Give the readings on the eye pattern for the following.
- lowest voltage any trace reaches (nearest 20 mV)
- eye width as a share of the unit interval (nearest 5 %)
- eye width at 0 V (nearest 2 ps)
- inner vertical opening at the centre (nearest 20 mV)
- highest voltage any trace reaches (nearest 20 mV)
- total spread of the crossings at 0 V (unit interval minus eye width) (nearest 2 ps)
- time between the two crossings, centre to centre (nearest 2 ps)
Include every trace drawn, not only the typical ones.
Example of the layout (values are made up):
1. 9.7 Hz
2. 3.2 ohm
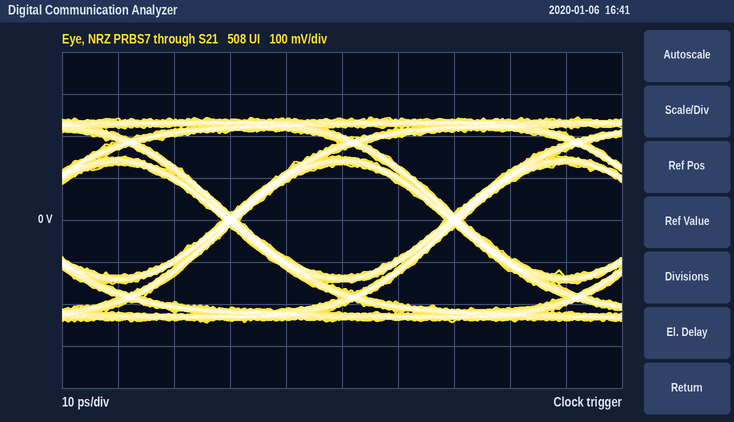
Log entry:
1. -240 mV
2. 90 %
3. 36 ps
4. 260 mV
5. 240 mV
6. 4 ps
7. 40 ps
